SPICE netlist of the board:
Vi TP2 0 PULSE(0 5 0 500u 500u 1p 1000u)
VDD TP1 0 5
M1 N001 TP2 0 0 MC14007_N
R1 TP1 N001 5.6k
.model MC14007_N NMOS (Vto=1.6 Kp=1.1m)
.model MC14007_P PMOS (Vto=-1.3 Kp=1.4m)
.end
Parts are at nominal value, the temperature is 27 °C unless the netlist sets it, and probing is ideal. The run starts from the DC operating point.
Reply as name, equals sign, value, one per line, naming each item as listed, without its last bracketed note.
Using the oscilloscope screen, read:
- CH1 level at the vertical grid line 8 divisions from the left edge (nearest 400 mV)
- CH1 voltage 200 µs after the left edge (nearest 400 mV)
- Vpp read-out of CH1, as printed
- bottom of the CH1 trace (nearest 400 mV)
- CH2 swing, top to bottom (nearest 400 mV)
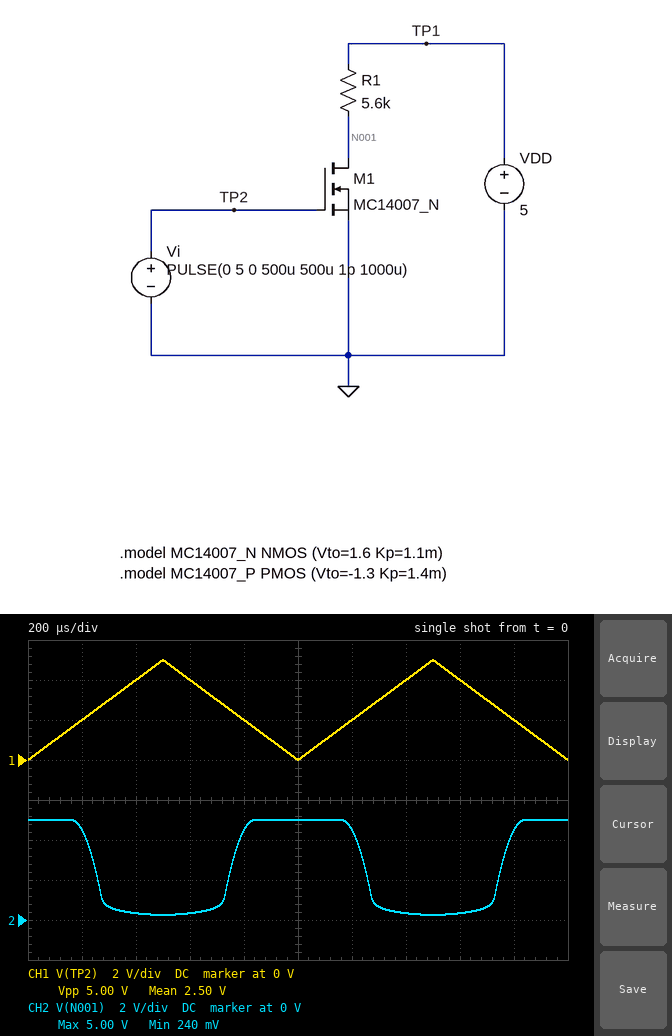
CH1 level at the vertical grid line 8 divisions from the left edge = 4.0 V
CH1 voltage 200 µs after the left edge = 2.0 V
Vpp read-out of CH1, as printed = 5.00 V
bottom of the CH1 trace = 0 V
CH2 swing, top to bottom = 4.8 V
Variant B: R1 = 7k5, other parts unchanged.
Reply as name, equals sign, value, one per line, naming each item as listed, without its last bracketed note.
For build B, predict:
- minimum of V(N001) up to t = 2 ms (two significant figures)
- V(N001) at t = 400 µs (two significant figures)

minimum of V(N001) up to t = 2 ms = 180 mV
V(N001) at t = 400 µs = 250 mV
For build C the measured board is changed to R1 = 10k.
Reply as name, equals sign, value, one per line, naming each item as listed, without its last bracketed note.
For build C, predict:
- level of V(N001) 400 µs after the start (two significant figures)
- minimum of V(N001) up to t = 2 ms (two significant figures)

level of V(N001) 400 µs after the start = 190 mV
minimum of V(N001) up to t = 2 ms = 130 mV
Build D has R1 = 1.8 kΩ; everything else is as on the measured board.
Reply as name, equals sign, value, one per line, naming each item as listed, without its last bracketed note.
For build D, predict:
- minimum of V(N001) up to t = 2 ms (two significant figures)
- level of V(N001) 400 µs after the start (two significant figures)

minimum of V(N001) up to t = 2 ms = 710 mV
level of V(N001) 400 µs after the start = 1.1 V
